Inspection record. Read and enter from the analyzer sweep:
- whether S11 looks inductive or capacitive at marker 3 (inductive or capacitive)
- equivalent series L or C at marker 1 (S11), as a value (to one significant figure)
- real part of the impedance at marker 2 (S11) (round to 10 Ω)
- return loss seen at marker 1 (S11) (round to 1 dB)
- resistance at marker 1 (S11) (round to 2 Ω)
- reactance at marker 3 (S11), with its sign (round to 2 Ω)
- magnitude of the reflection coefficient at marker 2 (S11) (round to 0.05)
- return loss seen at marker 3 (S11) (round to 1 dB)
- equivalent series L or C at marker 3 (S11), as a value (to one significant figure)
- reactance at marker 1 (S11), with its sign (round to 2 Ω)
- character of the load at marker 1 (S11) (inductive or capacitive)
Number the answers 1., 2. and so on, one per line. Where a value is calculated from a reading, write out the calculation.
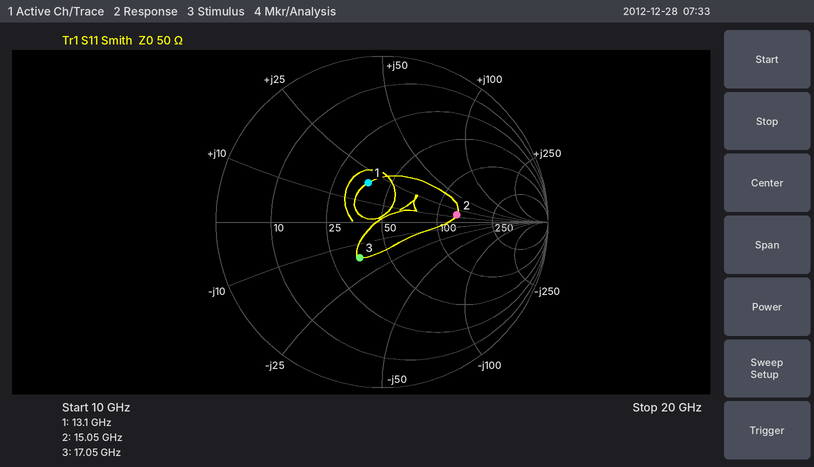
1. capacitive
2. L = 20 Ω/(2π × 13.1 GHz) ≈ 243 pH, so 200 pH to one significant figure
3. 130 Ω
4. 12 dB
5. 38 Ω
6. -16 Ω
7. 0.45
8. 12 dB
9. C = 1/(2π × 17.05 GHz × 16 Ω) ≈ 583 fF, so 600 fF to one significant figure
10. +20 Ω
11. inductive
